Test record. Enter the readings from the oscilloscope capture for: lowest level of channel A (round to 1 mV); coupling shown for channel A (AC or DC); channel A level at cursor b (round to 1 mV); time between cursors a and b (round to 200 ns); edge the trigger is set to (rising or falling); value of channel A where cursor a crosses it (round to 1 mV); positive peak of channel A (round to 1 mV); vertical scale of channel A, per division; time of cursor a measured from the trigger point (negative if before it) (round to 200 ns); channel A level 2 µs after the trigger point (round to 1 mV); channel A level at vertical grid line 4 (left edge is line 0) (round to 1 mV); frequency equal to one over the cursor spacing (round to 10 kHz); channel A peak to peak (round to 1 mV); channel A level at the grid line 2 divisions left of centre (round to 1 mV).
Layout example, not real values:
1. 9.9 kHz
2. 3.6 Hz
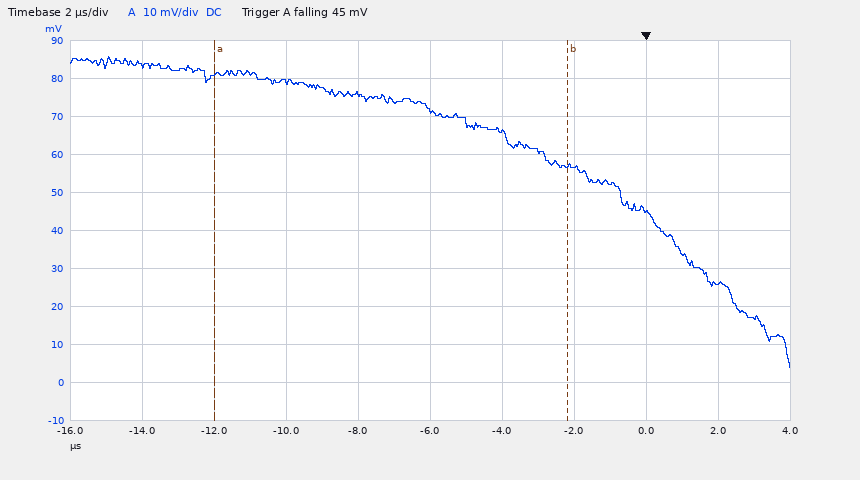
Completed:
1. 4 mV
2. DC
3. 57 mV
4. 9.8 µs
5. falling
6. 81 mV
7. 86 mV
8. 10 mV
9. -12.0 µs
10. 26 mV
11. 76 mV
12. 100 kHz
13. 82 mV
14. 79 mV
